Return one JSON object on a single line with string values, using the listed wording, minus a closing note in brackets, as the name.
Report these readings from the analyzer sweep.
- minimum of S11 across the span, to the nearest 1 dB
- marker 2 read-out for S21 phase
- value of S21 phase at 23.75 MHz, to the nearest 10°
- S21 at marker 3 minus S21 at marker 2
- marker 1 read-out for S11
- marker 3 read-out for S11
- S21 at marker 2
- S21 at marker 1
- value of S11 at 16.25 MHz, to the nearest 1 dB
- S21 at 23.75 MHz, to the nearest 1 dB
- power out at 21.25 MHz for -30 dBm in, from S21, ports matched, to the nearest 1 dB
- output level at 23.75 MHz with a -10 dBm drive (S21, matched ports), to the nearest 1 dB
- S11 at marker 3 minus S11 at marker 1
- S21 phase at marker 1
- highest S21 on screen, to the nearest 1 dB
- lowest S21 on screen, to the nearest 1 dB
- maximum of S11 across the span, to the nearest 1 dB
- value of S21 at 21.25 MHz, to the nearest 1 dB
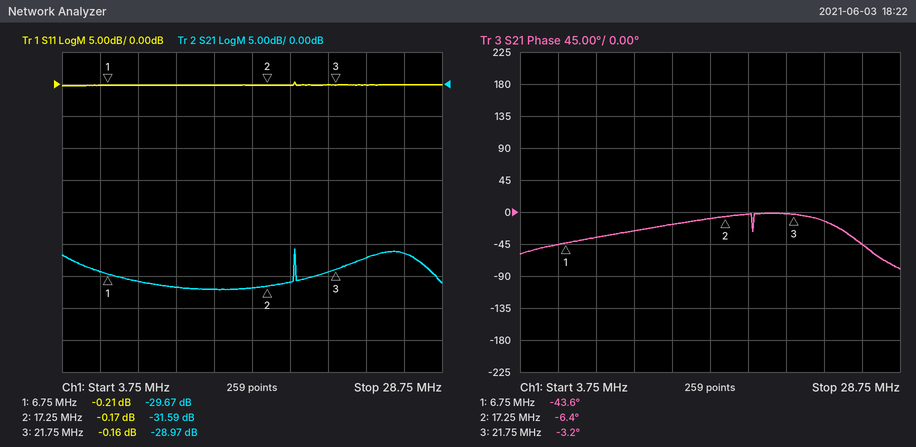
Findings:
{"minimum of S11 across the span, to the nearest 1 dB": "0 dB", "marker 2 read-out for S21 phase": "-6.4°", "value of S21 phase at 23.75 MHz, to the nearest 10°": "-10°", "S21 at marker 3 minus S21 at marker 2": "2.62 dB", "marker 1 read-out for S11": "-0.21 dB", "marker 3 read-out for S11": "-0.16 dB", "S21 at marker 2": "-31.59 dB", "S21 at marker 1": "-29.67 dB", "value of S11 at 16.25 MHz, to the nearest 1 dB": "0 dB", "S21 at 23.75 MHz, to the nearest 1 dB": "-27 dB", "power out at 21.25 MHz for -30 dBm in, from S21, ports matched, to the nearest 1 dB": "-59 dBm", "output level at 23.75 MHz with a -10 dBm drive (S21, matched ports), to the nearest 1 dB": "-37 dBm", "S11 at marker 3 minus S11 at marker 1": "0.05 dB", "S21 phase at marker 1": "-43.6°", "highest S21 on screen, to the nearest 1 dB": "-26 dB", "lowest S21 on screen, to the nearest 1 dB": "-32 dB", "maximum of S11 across the span, to the nearest 1 dB": "0 dB", "value of S21 at 21.25 MHz, to the nearest 1 dB": "-29 dB"}
